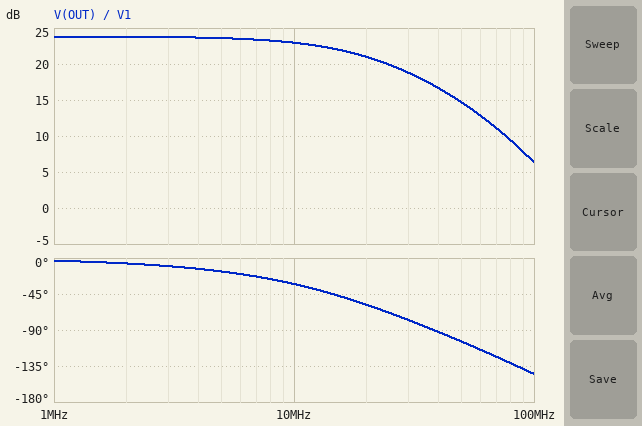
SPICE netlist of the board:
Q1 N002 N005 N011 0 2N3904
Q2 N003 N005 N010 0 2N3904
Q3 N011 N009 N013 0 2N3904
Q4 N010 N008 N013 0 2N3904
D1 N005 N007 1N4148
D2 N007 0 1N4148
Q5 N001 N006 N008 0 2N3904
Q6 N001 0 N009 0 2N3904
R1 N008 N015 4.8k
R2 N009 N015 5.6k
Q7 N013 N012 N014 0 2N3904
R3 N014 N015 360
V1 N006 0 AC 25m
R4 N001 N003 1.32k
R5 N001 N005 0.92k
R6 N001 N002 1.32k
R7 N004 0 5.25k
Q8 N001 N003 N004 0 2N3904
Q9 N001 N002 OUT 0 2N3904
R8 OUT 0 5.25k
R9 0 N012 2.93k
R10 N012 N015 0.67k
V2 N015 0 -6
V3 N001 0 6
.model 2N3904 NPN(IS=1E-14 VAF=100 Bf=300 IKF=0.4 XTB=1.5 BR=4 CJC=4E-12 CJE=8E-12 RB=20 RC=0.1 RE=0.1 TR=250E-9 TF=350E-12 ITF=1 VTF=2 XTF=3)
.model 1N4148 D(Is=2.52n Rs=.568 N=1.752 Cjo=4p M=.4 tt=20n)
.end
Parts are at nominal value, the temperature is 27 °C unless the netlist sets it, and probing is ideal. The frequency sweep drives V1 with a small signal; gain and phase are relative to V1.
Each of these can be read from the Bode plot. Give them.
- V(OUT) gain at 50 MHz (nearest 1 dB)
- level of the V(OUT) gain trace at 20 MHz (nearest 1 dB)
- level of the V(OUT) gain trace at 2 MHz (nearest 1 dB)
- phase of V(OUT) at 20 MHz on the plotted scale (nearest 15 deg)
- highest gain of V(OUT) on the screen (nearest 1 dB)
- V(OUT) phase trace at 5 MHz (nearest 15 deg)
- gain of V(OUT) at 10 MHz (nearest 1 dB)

15 dB
21 dB
24 dB
-60 deg
24 dB
-15 deg
23 dB
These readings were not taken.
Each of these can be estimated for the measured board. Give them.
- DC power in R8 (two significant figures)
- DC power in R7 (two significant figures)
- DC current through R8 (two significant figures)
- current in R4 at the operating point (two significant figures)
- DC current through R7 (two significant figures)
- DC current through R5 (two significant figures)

3.8 mW
4.0 mW
850 µA
580 µA
870 µA
5.1 mA
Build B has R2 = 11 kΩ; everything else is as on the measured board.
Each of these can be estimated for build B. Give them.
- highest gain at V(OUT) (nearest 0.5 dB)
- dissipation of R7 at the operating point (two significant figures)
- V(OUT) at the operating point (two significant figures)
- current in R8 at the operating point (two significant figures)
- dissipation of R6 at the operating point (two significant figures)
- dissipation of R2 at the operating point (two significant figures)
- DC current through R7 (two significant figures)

22.5 dB
4.5 mW
4.2 V
800 µA
1.0 mW
2.6 mW
920 µA
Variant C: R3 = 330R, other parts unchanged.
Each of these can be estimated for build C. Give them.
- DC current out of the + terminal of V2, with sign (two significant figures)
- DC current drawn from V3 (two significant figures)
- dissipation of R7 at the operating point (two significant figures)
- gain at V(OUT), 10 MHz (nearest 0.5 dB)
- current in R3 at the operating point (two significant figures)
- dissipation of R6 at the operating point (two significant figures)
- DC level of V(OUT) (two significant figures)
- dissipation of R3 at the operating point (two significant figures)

-5.1 mA
10 mA
3.9 mW
23.5 dB
1.4 mA
710 µW
4.4 V
620 µW
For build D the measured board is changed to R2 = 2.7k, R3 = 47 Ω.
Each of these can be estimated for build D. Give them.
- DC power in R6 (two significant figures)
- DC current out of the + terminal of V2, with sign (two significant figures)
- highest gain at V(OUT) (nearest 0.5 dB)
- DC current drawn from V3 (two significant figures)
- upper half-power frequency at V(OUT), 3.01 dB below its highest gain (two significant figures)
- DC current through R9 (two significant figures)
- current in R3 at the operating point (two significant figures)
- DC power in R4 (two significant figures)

12 mW
-13 mA
39.0 dB
16 mA
19 MHz
1.7 mA
8.3 mA
22 mW
